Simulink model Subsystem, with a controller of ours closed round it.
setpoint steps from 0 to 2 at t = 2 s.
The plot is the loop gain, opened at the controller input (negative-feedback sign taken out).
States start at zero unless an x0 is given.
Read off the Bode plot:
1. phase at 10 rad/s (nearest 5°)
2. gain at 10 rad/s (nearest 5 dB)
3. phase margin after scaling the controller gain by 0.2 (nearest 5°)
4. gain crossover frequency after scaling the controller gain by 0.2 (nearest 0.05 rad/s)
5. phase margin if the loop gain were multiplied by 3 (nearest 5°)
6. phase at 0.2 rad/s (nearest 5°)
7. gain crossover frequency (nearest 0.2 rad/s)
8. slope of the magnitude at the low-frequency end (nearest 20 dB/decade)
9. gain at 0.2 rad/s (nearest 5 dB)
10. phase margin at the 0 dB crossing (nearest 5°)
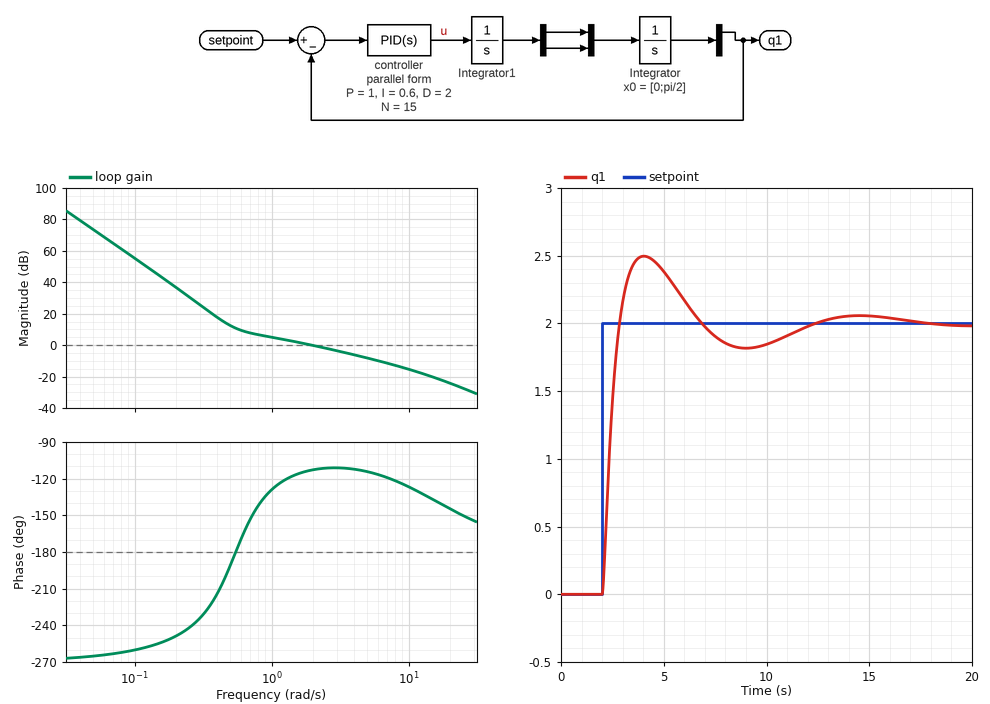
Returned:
-125°
-15 dB
-20°
0.45 rad/s
65°
-250°
2.0 rad/s
-60 dB/decade
35 dB
65°
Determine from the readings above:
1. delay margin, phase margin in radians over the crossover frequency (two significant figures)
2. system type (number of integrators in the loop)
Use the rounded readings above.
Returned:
0.57 s
3
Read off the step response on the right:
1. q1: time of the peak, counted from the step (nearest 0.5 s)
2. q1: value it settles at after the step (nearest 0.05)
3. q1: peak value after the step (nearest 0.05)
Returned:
2.0 s
2.00
2.50
